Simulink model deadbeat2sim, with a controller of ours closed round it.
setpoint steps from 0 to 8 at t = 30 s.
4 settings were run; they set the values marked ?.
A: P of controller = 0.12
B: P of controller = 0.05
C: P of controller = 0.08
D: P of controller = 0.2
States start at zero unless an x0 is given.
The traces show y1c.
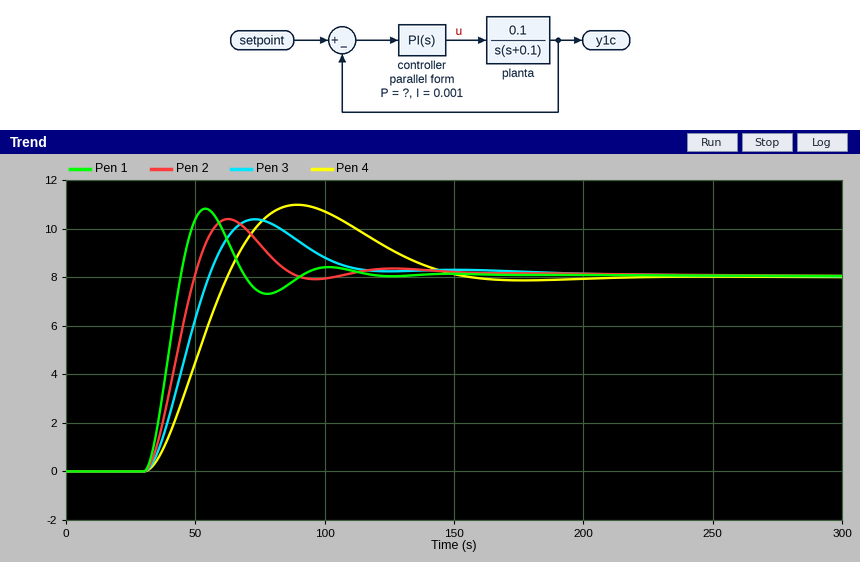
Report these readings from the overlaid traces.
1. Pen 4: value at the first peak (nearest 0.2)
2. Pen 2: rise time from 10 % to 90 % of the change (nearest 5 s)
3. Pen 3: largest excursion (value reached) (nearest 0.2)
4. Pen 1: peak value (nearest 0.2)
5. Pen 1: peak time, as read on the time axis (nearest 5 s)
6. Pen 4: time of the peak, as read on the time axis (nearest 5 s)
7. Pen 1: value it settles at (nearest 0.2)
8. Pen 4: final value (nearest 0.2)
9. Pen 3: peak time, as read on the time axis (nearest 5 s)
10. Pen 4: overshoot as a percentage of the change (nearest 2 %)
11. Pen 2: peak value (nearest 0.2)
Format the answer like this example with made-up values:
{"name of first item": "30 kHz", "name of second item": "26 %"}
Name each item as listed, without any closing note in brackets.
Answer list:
{"Pen 4: value at the first peak": "11.0", "Pen 2: rise time from 10 % to 90 % of the change": "15 s", "Pen 3: largest excursion (value reached)": "10.4", "Pen 1: peak value": "10.8", "Pen 1: peak time, as read on the time axis": "55 s", "Pen 4: time of the peak, as read on the time axis": "90 s", "Pen 1: value it settles at": "8.0", "Pen 4: final value": "8.0", "Pen 3: peak time, as read on the time axis": "75 s", "Pen 4: overshoot as a percentage of the change": "38 %", "Pen 2: peak value": "10.4"}
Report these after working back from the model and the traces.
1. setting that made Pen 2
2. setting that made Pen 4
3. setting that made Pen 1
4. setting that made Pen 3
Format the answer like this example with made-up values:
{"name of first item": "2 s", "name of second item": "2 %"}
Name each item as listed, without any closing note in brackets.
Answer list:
{"setting that made Pen 2": "A", "setting that made Pen 4": "B", "setting that made Pen 1": "D", "setting that made Pen 3": "C"}
